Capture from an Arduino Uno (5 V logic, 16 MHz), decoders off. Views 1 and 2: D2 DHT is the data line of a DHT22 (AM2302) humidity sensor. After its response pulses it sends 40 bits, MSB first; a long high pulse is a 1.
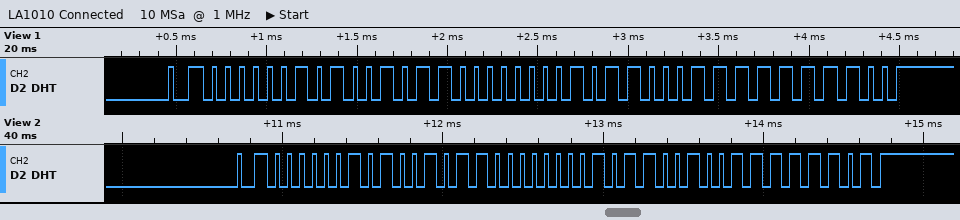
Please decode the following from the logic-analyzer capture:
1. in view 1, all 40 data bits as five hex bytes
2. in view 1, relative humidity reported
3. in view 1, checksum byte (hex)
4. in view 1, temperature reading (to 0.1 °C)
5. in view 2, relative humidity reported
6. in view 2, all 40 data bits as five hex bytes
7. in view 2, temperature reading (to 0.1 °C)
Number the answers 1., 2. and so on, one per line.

1. 02 96 01 63 FC
2. 66.2 %
3. 0xFC
4. 35.5 °C
5. 66.2 %
6. 02 96 01 64 FD
7. 35.6 °C
